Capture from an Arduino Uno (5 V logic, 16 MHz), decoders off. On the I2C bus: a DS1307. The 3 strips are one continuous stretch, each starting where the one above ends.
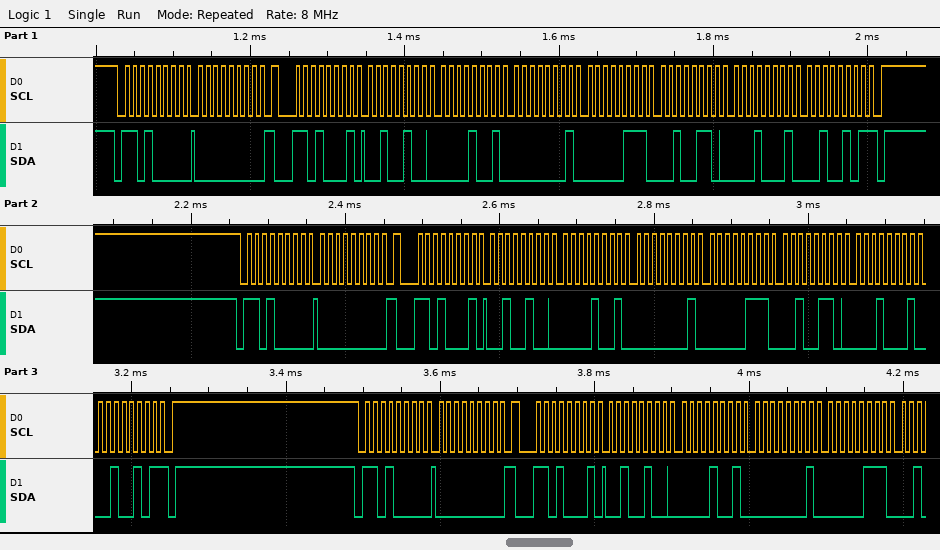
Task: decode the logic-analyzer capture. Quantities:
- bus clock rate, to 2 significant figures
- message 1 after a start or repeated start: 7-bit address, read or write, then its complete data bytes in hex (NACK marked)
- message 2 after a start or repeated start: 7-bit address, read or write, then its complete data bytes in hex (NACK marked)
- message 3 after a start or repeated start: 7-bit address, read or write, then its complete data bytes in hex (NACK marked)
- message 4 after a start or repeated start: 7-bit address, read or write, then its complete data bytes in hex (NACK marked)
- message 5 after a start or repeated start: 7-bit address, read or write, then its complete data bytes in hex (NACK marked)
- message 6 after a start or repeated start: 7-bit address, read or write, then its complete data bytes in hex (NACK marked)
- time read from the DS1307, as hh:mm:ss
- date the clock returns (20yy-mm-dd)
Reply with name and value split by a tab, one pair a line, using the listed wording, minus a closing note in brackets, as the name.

bus clock rate, to 2 significant figures	100 kHz
message 1 after a start or repeated start: 7-bit address, read or write, then its complete data bytes in hex	0x68 write: 00
message 2 after a start or repeated start: 7-bit address, read or write, then its complete data bytes in hex	0x68 read: 24 09 01 07 26 11 25 NACK
message 3 after a start or repeated start: 7-bit address, read or write, then its complete data bytes in hex	0x68 write: 00
message 4 after a start or repeated start: 7-bit address, read or write, then its complete data bytes in hex	0x68 read: 24 09 01 07 26 11 25 NACK
message 5 after a start or repeated start: 7-bit address, read or write, then its complete data bytes in hex	0x68 write: 00
message 6 after a start or repeated start: 7-bit address, read or write, then its complete data bytes in hex	0x68 read: 24 09 01 07
time read from the DS1307, as hh:mm:ss	01:09:24
date the clock returns	2025-11-26
